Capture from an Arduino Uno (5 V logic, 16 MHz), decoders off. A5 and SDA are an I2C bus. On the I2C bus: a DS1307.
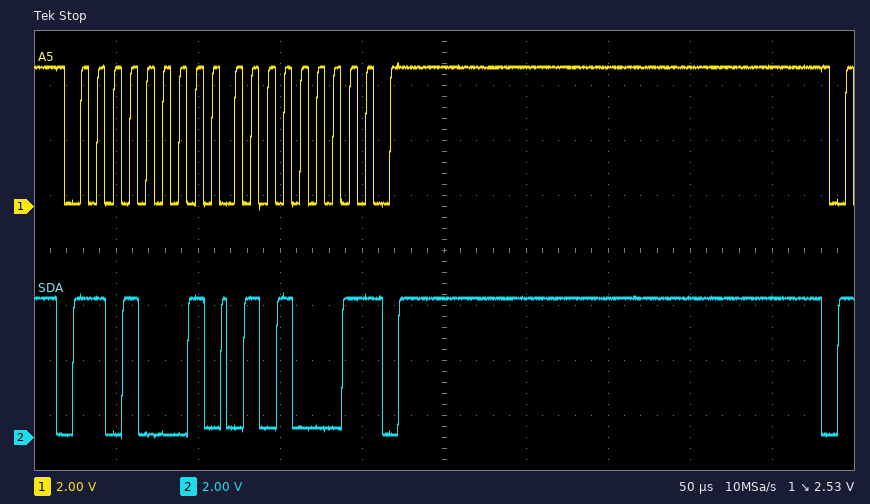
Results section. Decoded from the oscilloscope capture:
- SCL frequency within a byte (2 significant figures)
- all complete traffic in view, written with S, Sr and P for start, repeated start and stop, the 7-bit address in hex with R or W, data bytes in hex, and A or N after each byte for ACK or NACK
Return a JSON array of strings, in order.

["100 kHz", "S 68R A 51 N P"]
